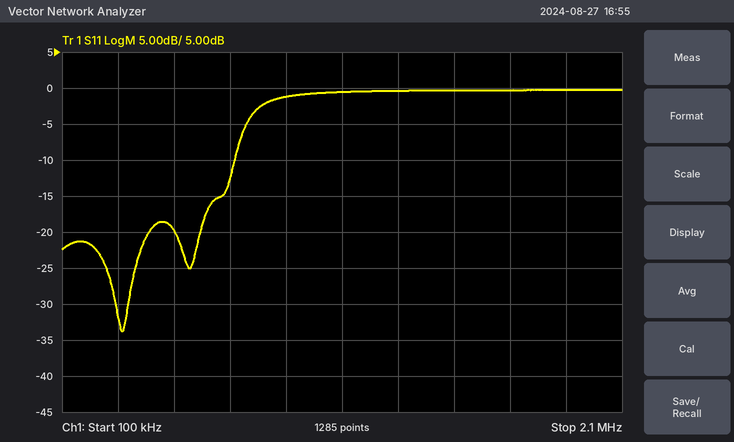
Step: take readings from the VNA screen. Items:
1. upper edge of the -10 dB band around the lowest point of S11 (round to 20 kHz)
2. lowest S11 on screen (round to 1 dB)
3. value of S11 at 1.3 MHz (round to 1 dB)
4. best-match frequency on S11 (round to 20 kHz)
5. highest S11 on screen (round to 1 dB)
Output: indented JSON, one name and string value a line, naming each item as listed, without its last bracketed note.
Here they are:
{
  "upper edge of the -10 dB band around the lowest point of S11": "720 kHz",
  "lowest S11 on screen": "-34 dB",
  "value of S11 at 1.3 MHz": "0 dB",
  "best-match frequency on S11": "320 kHz",
  "highest S11 on screen": "0 dB"
}
